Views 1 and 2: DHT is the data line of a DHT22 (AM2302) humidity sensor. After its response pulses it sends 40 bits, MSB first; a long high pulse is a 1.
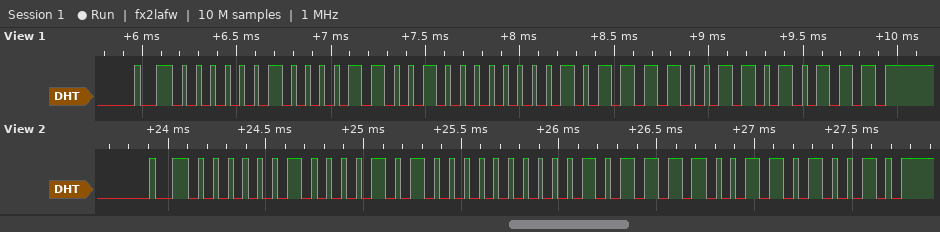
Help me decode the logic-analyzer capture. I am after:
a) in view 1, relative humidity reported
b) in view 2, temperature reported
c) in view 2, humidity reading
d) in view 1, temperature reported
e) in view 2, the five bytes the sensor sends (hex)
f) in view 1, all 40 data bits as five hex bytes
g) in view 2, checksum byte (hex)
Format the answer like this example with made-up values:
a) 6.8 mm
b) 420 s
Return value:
a) 53.7 %
b) 18.8 °C
c) 53.2 %
d) 18.8 °C
e) 02 14 00 BC D2
f) 02 19 00 BC D7
g) 0xD2
